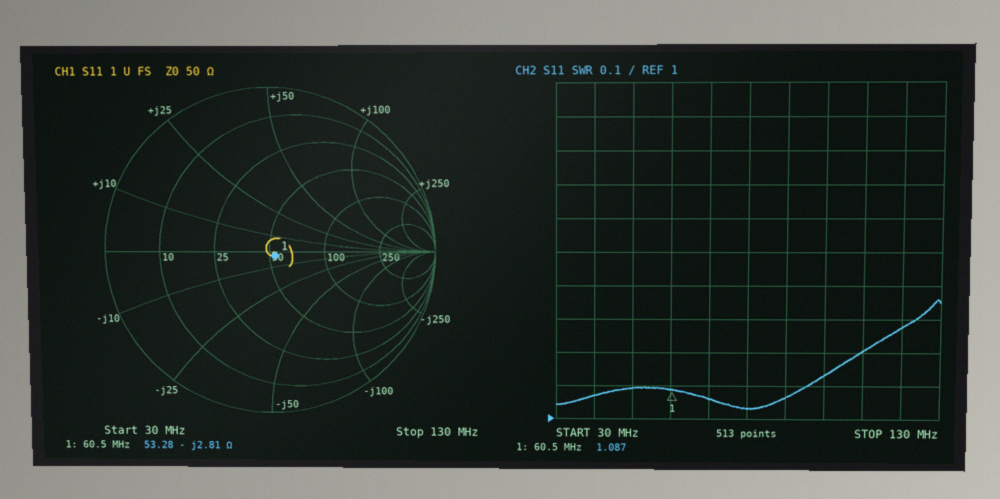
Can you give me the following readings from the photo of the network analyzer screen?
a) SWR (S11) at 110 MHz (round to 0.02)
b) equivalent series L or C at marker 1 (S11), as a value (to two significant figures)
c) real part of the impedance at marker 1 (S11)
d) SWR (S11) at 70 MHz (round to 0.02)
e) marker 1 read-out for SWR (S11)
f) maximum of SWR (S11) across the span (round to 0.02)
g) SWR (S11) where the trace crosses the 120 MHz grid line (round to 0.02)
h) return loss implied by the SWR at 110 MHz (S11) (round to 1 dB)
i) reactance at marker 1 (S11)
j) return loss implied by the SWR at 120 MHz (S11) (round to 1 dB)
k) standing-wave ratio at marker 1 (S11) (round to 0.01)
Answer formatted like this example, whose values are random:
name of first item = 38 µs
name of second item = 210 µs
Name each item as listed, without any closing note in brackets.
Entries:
SWR (S11) at 110 MHz = 1.20
equivalent series L or C at marker 1 (S11), as a value = 940 pF
real part of the impedance at marker 1 = 53.28 Ω
SWR (S11) at 70 MHz = 1.06
marker 1 read-out for SWR = 1.087
maximum of SWR (S11) across the span = 1.36
SWR (S11) where the trace crosses the 120 MHz grid line = 1.28
return loss implied by the SWR at 110 MHz (S11) = 21 dB
reactance at marker 1 = -2.81 Ω
return loss implied by the SWR at 120 MHz (S11) = 18 dB
standing-wave ratio at marker 1 (S11) = 1.09
